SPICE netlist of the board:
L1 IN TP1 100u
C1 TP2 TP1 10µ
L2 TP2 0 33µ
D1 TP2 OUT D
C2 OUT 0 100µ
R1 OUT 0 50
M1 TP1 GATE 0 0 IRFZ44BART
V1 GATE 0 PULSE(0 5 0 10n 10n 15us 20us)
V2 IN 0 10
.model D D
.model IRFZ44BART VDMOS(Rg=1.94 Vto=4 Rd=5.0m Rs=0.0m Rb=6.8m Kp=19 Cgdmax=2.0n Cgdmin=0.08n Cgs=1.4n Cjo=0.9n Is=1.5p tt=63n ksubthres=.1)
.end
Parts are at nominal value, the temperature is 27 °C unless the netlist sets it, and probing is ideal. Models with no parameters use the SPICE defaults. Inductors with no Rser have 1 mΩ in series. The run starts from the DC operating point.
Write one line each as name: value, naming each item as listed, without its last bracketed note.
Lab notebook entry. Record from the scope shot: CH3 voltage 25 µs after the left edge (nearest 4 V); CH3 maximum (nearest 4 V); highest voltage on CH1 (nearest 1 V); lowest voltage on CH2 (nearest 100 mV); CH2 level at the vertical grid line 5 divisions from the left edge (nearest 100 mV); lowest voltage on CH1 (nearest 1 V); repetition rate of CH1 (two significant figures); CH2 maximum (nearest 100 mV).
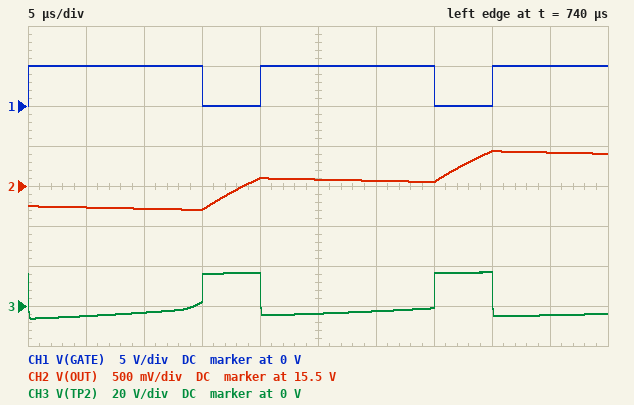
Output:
CH3 voltage 25 µs after the left edge: -4 V
CH3 maximum: 16 V
highest voltage on CH1: 5 V
lowest voltage on CH2: 15.2 V
CH2 level at the vertical grid line 5 divisions from the left edge: 15.6 V
lowest voltage on CH1: 0 V
repetition rate of CH1: 50 kHz
CH2 maximum: 15.9 V
